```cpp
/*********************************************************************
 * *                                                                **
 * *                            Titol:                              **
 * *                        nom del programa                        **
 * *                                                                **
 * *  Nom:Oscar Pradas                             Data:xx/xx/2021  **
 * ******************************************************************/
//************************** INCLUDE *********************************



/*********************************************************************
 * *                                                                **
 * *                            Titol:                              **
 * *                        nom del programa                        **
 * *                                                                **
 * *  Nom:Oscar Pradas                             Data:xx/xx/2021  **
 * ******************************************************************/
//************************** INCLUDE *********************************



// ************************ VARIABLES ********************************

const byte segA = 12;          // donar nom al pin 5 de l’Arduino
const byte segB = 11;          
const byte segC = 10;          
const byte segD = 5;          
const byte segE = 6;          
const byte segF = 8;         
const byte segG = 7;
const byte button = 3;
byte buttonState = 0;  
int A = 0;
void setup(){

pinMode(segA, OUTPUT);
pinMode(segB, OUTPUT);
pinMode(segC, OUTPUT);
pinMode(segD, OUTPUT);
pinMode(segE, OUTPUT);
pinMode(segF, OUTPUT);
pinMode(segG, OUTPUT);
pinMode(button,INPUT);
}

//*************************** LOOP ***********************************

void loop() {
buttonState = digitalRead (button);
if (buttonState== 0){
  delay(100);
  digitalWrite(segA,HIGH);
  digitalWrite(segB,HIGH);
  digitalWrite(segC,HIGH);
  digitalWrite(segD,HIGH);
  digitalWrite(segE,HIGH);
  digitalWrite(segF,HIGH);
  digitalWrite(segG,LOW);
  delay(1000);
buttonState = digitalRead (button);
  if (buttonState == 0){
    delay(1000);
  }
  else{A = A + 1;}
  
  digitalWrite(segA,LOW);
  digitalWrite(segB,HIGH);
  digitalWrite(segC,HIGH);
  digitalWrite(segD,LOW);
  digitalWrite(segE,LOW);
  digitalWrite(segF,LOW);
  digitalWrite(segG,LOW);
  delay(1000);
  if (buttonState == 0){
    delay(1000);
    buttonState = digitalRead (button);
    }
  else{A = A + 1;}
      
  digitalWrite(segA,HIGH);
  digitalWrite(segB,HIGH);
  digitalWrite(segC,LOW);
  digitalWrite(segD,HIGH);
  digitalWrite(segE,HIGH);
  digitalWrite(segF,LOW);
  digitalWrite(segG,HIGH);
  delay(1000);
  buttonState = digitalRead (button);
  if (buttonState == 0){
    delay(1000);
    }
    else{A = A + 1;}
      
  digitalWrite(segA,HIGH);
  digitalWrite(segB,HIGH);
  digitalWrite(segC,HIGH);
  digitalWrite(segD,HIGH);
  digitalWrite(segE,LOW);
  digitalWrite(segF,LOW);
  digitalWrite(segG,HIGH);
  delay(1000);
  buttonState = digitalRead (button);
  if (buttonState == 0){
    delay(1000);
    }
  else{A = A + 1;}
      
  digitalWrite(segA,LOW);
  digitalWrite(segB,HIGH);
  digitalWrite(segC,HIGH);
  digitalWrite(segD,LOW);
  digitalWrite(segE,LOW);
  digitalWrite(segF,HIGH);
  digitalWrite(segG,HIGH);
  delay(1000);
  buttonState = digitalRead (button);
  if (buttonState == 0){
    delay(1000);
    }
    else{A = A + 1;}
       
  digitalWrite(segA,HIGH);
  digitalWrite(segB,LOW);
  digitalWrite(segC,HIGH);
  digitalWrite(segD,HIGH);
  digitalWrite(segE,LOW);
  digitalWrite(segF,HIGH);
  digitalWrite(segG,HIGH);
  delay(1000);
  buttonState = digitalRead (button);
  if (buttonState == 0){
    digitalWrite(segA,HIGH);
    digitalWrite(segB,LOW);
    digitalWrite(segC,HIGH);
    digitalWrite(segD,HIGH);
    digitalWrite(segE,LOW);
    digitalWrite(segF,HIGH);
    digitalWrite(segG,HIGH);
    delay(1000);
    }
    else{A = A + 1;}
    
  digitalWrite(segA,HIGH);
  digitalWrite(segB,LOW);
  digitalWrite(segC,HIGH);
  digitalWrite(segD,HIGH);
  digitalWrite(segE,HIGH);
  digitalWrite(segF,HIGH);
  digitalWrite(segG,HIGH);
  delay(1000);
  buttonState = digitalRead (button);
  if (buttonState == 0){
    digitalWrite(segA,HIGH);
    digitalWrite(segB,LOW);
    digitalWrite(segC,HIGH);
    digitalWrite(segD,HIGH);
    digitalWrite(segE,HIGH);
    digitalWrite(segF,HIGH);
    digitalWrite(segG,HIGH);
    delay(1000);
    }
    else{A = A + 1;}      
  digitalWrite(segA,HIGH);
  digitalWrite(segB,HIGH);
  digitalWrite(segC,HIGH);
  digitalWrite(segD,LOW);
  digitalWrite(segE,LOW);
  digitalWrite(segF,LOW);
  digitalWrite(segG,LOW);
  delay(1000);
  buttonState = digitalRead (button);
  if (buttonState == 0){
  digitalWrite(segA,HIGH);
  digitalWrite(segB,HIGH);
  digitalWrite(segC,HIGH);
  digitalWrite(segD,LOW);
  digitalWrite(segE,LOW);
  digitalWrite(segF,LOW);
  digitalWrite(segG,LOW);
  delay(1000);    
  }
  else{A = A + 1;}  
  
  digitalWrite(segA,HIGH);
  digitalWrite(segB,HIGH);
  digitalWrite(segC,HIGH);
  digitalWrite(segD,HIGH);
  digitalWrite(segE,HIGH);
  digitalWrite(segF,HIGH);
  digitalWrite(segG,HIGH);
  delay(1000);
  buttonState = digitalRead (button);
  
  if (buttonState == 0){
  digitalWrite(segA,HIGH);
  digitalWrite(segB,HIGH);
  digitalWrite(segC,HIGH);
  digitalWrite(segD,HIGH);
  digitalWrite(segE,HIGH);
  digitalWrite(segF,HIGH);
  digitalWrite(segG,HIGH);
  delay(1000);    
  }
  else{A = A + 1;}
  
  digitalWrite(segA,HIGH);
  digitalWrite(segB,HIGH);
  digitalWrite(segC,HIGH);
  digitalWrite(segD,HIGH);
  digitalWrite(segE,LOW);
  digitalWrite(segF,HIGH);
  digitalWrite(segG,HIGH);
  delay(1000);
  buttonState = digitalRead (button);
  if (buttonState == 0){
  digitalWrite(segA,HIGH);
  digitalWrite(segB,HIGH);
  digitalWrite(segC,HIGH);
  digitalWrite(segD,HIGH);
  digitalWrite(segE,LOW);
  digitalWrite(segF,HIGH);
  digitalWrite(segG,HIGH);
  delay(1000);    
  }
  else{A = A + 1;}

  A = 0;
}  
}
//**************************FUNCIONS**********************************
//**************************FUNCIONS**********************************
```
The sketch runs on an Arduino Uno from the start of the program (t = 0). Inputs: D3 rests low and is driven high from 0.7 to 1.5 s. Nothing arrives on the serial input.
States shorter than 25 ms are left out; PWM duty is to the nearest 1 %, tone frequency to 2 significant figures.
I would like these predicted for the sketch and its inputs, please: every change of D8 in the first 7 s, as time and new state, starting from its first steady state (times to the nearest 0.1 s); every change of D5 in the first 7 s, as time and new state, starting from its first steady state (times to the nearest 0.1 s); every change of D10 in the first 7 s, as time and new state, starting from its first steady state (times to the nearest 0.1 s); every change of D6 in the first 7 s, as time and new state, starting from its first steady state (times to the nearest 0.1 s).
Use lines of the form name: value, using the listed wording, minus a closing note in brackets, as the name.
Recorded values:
every change of D8 in the first 7 s, as time and new state, starting from its first steady state: 0 s low; 0.1 s high; 1.1 s low; 6.1 s high
every change of D5 in the first 7 s, as time and new state, starting from its first steady state: 0 s low; 0.1 s high; 1.1 s low; 2.1 s high; 6.1 s low
every change of D10 in the first 7 s, as time and new state, starting from its first steady state: 0 s low; 0.1 s high; 2.1 s low; 4.1 s high
every change of D6 in the first 7 s, as time and new state, starting from its first steady state: 0 s low; 0.1 s high; 1.1 s low; 2.1 s high; 4.1 s low
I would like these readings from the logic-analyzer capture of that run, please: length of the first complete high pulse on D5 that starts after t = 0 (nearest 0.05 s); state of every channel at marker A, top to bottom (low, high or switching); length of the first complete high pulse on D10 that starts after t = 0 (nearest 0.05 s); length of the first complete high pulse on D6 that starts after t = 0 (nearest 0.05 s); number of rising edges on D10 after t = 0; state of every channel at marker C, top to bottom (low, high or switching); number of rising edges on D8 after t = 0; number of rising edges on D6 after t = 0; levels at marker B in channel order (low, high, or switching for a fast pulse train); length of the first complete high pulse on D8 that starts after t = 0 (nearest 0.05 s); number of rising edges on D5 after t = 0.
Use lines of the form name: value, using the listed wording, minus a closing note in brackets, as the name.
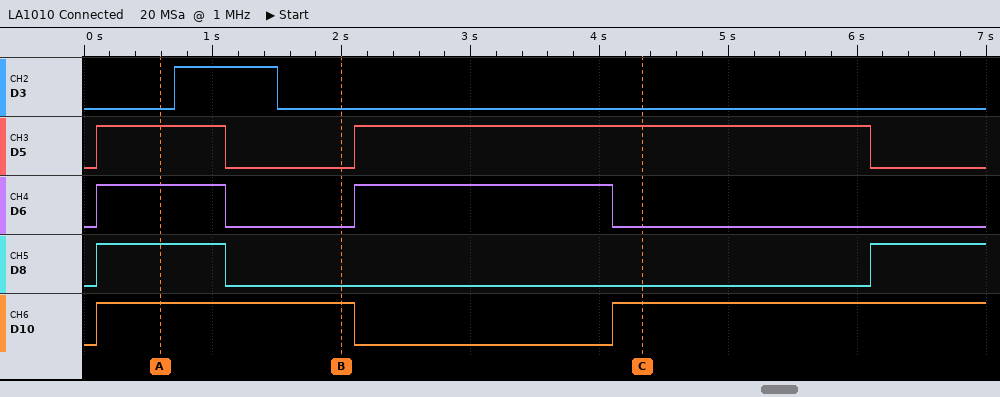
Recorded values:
length of the first complete high pulse on D5 that starts after t = 0: 1.00 s
state of every channel at marker A, top to bottom: D3 low, D5 high, D6 high, D8 high, D10 high
length of the first complete high pulse on D10 that starts after t = 0: 2.00 s
length of the first complete high pulse on D6 that starts after t = 0: 1.00 s
number of rising edges on D10 after t = 0: 2
state of every channel at marker C, top to bottom: D3 low, D5 high, D6 low, D8 low, D10 high
number of rising edges on D8 after t = 0: 2
number of rising edges on D6 after t = 0: 2
levels at marker B in channel order: D3 low, D5 low, D6 low, D8 low, D10 high
length of the first complete high pulse on D8 that starts after t = 0: 1.00 s
number of rising edges on D5 after t = 0: 2
